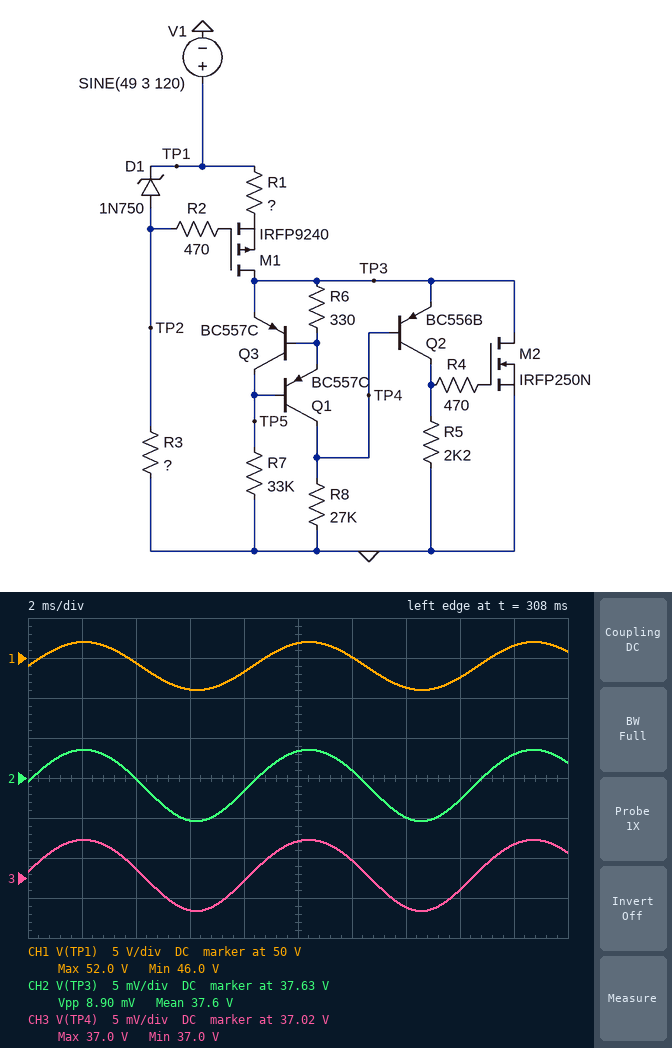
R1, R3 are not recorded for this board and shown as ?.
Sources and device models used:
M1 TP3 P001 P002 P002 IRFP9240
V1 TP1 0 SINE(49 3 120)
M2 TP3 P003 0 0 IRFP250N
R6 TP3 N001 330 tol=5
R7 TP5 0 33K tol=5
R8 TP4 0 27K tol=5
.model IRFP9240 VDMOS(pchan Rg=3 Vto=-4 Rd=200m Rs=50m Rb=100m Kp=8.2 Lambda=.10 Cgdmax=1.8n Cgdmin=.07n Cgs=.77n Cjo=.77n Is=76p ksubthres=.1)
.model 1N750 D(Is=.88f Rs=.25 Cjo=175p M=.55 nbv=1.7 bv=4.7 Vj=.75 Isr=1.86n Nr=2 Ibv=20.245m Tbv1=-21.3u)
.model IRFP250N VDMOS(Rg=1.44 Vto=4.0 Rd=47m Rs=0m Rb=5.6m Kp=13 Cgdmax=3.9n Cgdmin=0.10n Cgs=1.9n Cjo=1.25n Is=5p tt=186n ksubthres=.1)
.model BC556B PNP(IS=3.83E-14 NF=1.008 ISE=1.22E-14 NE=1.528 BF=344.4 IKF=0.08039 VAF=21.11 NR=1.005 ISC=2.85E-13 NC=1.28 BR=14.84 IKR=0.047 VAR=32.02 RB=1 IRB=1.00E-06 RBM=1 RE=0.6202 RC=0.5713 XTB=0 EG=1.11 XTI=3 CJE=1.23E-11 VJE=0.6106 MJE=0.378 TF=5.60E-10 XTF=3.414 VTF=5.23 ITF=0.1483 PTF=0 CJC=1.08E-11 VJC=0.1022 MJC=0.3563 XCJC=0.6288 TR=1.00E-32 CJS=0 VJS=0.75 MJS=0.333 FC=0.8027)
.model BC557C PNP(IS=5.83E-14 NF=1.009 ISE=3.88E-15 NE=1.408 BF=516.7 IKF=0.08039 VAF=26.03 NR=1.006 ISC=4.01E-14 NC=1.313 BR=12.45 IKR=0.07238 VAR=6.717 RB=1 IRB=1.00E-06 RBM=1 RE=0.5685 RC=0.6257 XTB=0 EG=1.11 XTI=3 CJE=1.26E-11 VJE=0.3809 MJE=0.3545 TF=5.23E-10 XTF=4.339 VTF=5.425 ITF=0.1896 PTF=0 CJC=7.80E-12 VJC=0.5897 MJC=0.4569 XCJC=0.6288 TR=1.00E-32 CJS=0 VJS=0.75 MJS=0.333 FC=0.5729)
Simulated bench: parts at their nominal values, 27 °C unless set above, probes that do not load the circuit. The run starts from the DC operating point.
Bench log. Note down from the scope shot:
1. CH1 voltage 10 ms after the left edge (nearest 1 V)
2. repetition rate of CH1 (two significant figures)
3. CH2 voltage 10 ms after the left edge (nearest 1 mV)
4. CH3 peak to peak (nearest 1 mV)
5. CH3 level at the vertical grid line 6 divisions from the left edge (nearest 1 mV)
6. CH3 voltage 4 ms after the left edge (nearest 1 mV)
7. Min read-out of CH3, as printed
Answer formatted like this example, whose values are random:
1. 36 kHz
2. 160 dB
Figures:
1. 52 V
2. 120 Hz
3. 37.638 V
4. 9 mV
5. 37.017 V
6. 37.016 V
7. 37.0 V
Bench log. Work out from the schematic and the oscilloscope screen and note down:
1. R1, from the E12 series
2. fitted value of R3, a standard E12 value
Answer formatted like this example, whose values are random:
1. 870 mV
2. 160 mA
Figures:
1. 4.7 Ω
2. 2.2 kΩ
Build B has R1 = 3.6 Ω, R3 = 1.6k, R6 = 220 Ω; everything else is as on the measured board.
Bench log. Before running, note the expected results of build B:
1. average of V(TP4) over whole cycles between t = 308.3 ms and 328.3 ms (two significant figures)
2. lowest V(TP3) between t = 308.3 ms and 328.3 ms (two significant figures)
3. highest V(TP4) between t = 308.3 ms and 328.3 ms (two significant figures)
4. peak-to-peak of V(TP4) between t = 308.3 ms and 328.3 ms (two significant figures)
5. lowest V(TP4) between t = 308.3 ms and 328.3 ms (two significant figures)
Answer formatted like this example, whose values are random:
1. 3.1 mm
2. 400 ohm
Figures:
1. 48 V
2. 46 V
3. 49 V
4. 3.5 V
5. 45 V
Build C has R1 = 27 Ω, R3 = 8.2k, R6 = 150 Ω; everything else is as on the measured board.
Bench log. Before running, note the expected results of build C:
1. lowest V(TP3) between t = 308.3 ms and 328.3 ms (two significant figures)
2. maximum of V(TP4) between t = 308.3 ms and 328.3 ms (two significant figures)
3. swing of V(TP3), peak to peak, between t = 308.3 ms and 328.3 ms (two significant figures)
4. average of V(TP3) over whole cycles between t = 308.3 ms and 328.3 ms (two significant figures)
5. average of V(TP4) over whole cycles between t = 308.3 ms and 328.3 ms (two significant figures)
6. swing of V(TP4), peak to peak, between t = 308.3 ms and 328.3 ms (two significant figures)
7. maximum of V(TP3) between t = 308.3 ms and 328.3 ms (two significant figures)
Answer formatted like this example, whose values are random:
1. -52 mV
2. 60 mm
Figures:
1. 46 V
2. 51 V
3. 6.0 V
4. 49 V
5. 48 V
6. 5.9 V
7. 52 V
